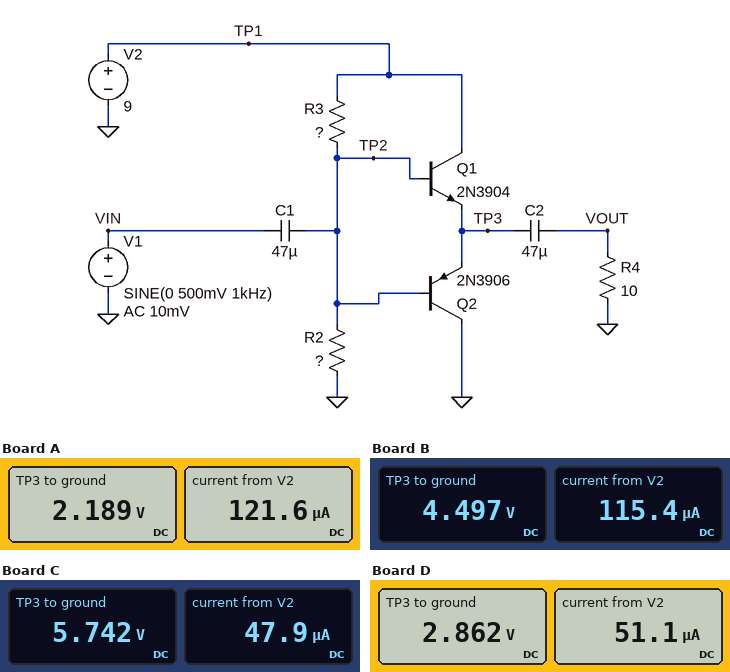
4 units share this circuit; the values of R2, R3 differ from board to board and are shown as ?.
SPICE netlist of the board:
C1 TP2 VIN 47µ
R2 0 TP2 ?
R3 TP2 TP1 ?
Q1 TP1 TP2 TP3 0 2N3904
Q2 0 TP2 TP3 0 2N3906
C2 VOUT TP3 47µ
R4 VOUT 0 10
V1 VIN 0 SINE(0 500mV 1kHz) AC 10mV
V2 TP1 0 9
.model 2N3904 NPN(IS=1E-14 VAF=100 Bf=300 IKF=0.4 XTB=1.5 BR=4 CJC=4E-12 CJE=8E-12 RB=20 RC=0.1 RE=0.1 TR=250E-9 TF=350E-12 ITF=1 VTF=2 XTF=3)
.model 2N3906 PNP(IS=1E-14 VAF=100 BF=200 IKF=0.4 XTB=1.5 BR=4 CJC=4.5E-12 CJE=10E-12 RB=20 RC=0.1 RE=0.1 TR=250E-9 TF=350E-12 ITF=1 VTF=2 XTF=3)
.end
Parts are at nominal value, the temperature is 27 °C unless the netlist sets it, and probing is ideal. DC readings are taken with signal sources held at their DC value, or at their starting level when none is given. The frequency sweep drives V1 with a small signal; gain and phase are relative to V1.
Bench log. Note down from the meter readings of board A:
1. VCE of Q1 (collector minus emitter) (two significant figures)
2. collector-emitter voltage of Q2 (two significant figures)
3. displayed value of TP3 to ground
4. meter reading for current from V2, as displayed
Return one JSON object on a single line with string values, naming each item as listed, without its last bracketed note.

{"VCE of Q1 (collector minus emitter)": "6.8 V", "collector-emitter voltage of Q2": "-2.2 V", "displayed value of TP3 to ground": "2.189 V", "meter reading for current from V2, as displayed": "121.6 µA"}
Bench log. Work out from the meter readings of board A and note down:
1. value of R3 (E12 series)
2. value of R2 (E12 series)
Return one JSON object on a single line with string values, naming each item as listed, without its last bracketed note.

{"value of R3": "56 kΩ", "value of R2": "18 kΩ"}
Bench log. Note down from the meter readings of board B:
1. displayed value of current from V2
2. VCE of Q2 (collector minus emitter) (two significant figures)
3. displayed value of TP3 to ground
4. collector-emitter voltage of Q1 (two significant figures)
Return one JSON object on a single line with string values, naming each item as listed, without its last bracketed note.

{"displayed value of current from V2": "115.4 µA", "VCE of Q2 (collector minus emitter)": "-4.5 V", "displayed value of TP3 to ground": "4.497 V", "collector-emitter voltage of Q1": "4.5 V"}
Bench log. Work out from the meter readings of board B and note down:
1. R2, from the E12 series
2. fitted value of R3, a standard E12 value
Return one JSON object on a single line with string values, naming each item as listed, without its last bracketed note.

{"R2, from the E12 series": "39 kΩ", "fitted value of R3, a standard E12 value": "39 kΩ"}
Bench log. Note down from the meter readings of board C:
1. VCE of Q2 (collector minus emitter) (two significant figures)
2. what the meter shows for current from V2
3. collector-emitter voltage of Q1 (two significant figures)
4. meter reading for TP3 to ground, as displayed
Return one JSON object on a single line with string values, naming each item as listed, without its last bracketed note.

{"VCE of Q2 (collector minus emitter)": "-5.7 V", "what the meter shows for current from V2": "47.9 µA", "collector-emitter voltage of Q1": "3.3 V", "meter reading for TP3 to ground, as displayed": "5.742 V"}
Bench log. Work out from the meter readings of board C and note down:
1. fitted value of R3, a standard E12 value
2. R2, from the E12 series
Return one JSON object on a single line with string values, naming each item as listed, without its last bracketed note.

{"fitted value of R3, a standard E12 value": "68 kΩ", "R2, from the E12 series": "120 kΩ"}
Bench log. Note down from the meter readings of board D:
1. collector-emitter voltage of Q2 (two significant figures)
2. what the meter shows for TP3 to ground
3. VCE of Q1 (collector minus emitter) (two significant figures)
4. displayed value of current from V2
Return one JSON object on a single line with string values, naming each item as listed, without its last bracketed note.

{"collector-emitter voltage of Q2": "-2.9 V", "what the meter shows for TP3 to ground": "2.862 V", "VCE of Q1 (collector minus emitter)": "6.1 V", "displayed value of current from V2": "51.1 µA"}
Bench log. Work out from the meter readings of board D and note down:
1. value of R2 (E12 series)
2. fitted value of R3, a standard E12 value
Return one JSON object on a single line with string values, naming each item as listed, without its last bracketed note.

{"value of R2": "56 kΩ", "fitted value of R3, a standard E12 value": "120 kΩ"}
